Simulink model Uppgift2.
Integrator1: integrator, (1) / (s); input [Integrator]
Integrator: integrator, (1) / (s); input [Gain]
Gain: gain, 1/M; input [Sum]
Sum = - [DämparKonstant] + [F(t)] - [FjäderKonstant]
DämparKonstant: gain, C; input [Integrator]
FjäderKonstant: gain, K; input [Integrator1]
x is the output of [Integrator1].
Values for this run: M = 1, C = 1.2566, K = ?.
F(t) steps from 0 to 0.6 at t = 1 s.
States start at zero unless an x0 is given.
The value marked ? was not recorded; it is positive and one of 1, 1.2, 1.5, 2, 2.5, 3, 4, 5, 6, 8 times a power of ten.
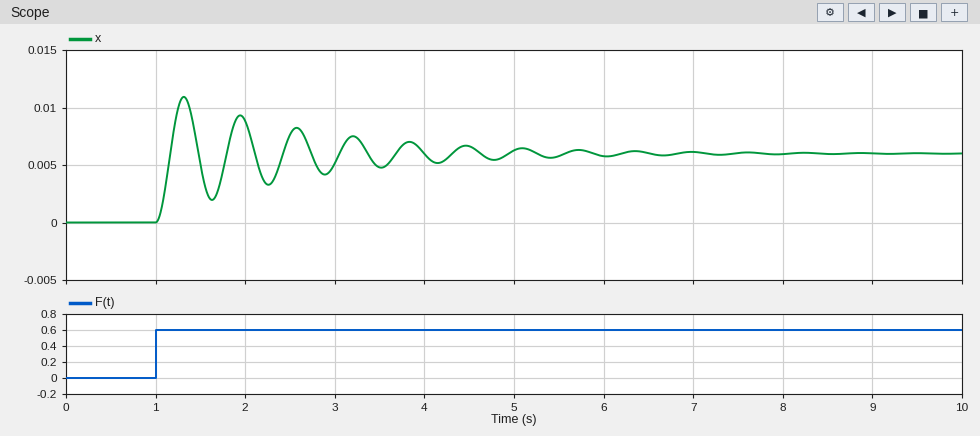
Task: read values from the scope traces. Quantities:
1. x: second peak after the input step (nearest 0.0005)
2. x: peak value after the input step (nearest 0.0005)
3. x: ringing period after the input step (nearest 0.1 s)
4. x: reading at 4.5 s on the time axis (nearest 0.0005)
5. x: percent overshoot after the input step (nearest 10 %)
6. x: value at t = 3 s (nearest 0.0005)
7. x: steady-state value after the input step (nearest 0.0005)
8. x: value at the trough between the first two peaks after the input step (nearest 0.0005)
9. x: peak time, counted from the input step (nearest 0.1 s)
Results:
0.0095
0.0110
0.6 s
0.0065
80 %
0.0050
0.0060
0.0020
0.3 s
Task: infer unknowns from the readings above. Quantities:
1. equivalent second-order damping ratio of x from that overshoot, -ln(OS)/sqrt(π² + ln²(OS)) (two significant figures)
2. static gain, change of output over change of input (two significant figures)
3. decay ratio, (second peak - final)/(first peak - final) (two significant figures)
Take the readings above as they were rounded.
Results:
0.071
0.010
0.70
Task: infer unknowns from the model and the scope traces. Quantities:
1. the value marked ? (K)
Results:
100
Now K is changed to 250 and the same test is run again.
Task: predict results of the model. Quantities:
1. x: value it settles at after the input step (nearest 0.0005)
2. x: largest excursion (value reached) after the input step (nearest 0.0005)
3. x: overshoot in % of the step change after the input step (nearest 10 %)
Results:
0.0025
0.0045
90 %
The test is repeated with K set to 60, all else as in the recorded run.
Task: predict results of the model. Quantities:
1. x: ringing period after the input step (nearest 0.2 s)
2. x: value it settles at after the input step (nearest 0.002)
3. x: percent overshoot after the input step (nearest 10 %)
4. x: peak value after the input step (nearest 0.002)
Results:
0.8 s
0.010
80 %
0.018
